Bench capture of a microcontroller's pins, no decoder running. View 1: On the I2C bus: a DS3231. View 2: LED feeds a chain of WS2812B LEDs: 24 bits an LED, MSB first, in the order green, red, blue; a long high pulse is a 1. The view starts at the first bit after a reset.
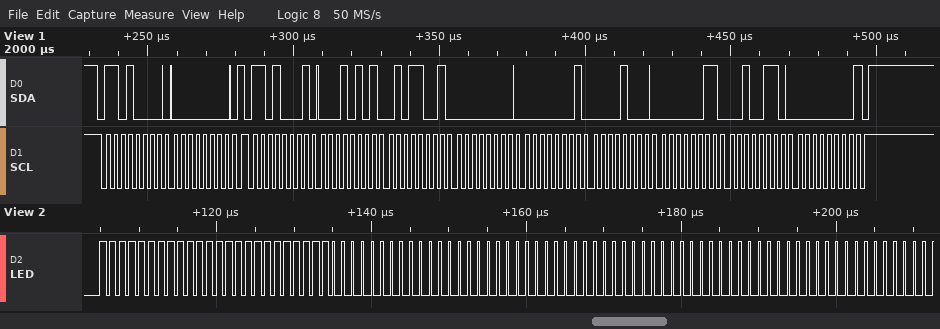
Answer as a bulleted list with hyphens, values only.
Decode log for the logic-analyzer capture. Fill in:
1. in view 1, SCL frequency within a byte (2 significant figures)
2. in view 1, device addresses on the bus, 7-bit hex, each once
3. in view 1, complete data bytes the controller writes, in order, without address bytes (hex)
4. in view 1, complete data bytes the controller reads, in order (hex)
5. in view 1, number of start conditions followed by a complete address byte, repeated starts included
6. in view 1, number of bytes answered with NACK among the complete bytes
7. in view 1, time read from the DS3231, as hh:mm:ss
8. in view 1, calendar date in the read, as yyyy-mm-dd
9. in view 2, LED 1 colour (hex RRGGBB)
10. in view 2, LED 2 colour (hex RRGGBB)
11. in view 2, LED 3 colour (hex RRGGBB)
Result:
- 400 kHz
- 0x68
- 00
- 15 59 00 01 08 03 26 00
- 2
- 1
- 00:59:15
- 2026-03-08
- #FFFFFF
- #000000
- #000000
